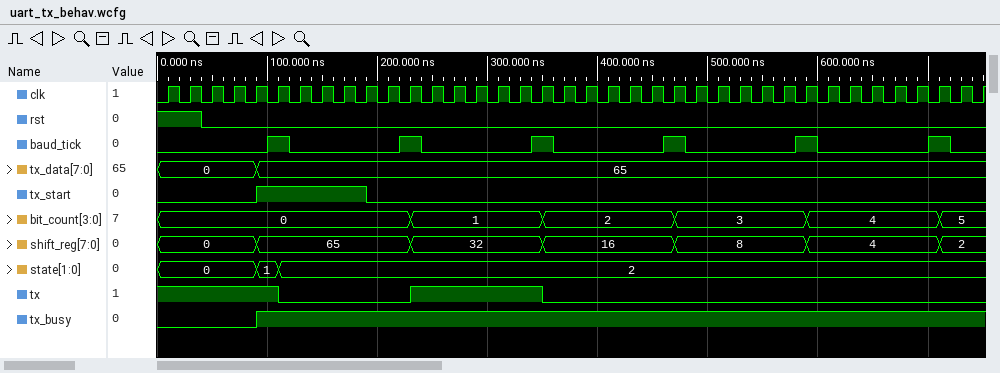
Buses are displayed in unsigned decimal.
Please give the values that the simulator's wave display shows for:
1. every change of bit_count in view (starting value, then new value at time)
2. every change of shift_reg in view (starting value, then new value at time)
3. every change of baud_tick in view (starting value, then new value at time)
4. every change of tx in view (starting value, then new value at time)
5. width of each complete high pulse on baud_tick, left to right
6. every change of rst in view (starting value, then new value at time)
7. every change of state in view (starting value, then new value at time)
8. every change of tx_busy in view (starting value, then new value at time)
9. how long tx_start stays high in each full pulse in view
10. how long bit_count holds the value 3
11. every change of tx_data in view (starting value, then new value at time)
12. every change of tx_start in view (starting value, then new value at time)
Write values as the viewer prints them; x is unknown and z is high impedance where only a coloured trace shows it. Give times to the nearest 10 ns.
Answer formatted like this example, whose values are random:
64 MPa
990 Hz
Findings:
0, 1 at 230 ns, 2 at 350 ns, 3 at 470 ns, 4 at 590 ns, 5 at 710 ns
0, 65 at 90 ns, 32 at 230 ns, 16 at 350 ns, 8 at 470 ns, 4 at 590 ns, 2 at 710 ns
0, 1 at 100 ns, 0 at 120 ns, 1 at 220 ns, 0 at 240 ns, 1 at 340 ns, 0 at 360 ns, 1 at 460 ns, 0 at 480 ns, 1 at 580 ns, 0 at 600 ns, 1 at 700 ns, 0 at 720 ns
1, 0 at 110 ns, 1 at 230 ns, 0 at 350 ns
20 ns, 20 ns, 20 ns, 20 ns, 20 ns, 20 ns
1, 0 at 40 ns
0, 1 at 90 ns, 2 at 110 ns
0, 1 at 90 ns
100 ns
120 ns
0, 65 at 90 ns
0, 1 at 90 ns, 0 at 190 ns
